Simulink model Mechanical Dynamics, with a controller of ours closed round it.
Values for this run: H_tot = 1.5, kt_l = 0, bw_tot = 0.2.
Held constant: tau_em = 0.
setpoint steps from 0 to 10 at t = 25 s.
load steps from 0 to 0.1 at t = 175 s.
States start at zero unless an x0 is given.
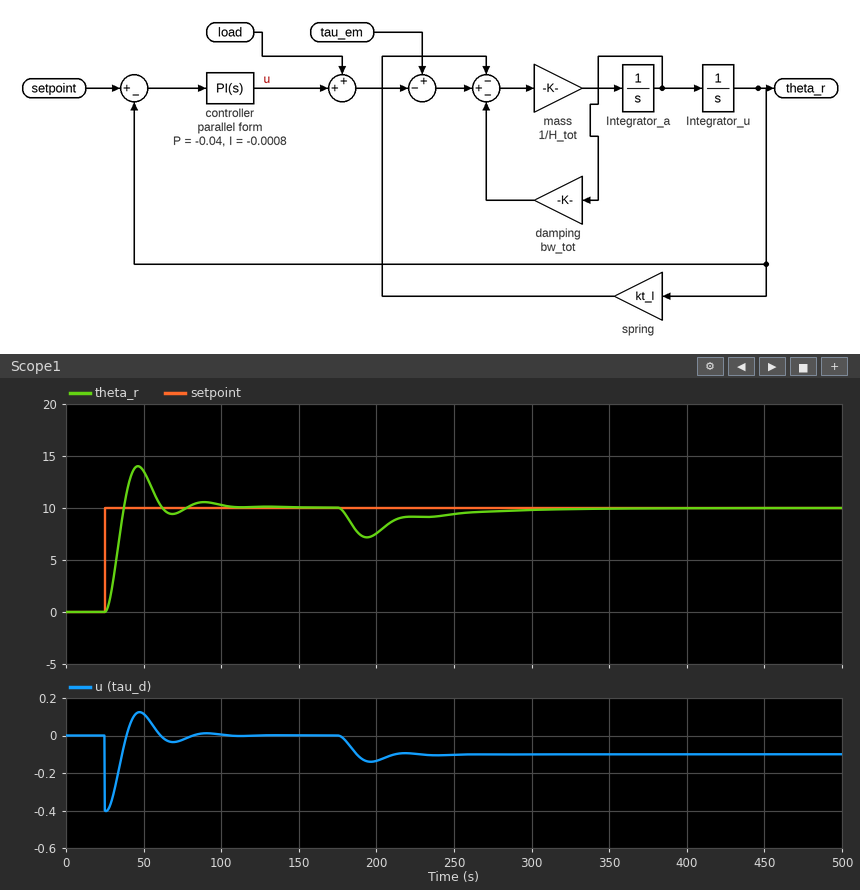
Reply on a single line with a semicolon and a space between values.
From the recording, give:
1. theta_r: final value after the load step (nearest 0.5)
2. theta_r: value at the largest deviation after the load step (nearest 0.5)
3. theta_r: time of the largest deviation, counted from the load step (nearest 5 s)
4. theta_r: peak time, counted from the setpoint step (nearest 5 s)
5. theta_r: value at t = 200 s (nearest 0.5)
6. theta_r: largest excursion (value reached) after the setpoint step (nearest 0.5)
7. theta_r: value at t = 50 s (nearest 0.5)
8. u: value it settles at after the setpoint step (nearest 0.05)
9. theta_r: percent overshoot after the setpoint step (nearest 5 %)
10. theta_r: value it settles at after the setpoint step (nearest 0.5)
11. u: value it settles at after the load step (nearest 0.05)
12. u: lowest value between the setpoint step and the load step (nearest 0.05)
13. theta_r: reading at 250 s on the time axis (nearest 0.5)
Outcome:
10.0; 7.0; 20 s; 20 s; 7.5; 14.0; 13.5; 0.00; 40 %; 10.0; -0.10; -0.40; 9.5
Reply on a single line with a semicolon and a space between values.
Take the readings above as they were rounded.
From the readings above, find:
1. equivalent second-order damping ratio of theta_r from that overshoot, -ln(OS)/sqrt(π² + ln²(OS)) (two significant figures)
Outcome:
0.28
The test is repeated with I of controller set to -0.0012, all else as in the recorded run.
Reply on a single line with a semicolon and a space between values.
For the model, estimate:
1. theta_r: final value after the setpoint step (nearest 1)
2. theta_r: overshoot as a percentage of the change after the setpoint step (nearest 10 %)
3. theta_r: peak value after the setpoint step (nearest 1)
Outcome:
10; 50 %; 15
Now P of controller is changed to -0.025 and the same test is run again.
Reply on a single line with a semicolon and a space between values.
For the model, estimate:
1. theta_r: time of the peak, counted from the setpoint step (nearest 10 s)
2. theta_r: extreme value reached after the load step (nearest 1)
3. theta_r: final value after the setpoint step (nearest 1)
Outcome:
30 s; 6; 10
